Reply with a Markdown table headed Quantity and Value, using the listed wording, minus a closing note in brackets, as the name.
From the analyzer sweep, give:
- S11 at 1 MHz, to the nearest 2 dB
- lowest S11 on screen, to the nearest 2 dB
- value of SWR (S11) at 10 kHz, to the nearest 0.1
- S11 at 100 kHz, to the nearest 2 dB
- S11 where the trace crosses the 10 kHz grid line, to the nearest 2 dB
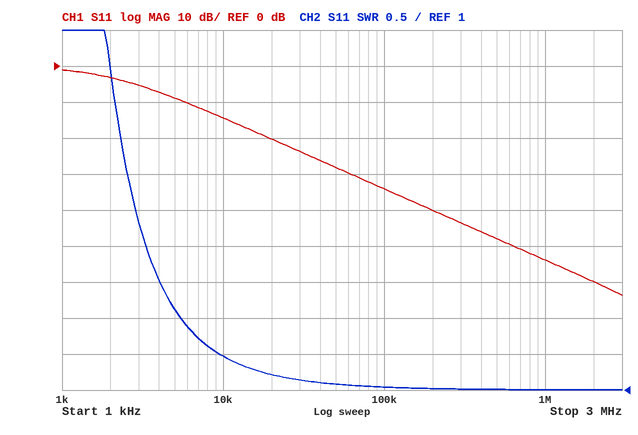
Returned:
| Quantity | Value |
|---|---|
| S11 at 1 MHz, to the nearest 2 dB | -54 dB |
| lowest S11 on screen, to the nearest 2 dB | -64 dB |
| value of SWR (S11) at 10 kHz, to the nearest 0.1 | 1.5 |
| S11 at 100 kHz, to the nearest 2 dB | -34 dB |
| S11 where the trace crosses the 10 kHz grid line, to the nearest 2 dB | -14 dB |
